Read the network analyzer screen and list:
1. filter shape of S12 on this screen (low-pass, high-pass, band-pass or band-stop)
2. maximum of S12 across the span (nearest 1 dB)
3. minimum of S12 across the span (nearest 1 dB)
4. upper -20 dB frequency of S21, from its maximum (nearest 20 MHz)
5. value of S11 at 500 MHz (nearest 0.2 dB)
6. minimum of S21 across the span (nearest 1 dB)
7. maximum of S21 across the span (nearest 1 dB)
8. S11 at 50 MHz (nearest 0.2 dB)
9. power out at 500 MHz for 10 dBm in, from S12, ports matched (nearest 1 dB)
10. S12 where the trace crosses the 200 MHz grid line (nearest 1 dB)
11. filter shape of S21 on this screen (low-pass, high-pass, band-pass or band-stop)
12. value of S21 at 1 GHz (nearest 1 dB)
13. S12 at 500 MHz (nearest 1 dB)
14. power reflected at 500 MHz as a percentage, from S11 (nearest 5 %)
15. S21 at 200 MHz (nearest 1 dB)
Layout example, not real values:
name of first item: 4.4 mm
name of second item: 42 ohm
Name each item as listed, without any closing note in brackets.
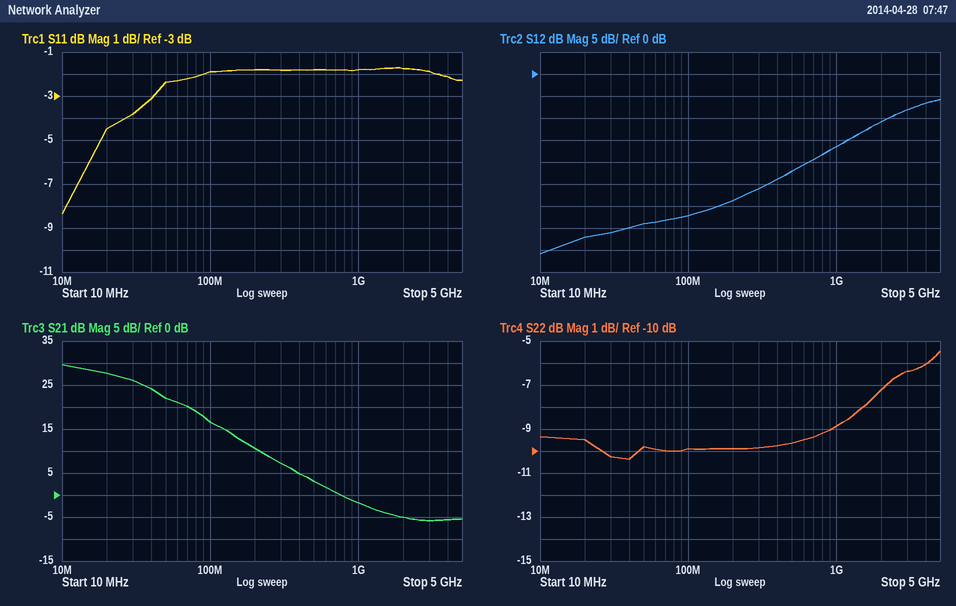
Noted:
filter shape of S12 on this screen: high-pass
maximum of S12 across the span: -6 dB
minimum of S12 across the span: -41 dB
upper -20 dB frequency of S21, from its maximum: 220 MHz
value of S11 at 500 MHz: -1.8 dB
minimum of S21 across the span: -6 dB
maximum of S21 across the span: 30 dB
S11 at 50 MHz: -2.4 dB
power out at 500 MHz for 10 dBm in, from S12, ports matched: -12 dBm
S12 where the trace crosses the 200 MHz grid line: -29 dB
filter shape of S21 on this screen: low-pass
value of S21 at 1 GHz: -2 dB
S12 at 500 MHz: -22 dB
power reflected at 500 MHz as a percentage, from S11: 65 %
S21 at 200 MHz: 11 dB
